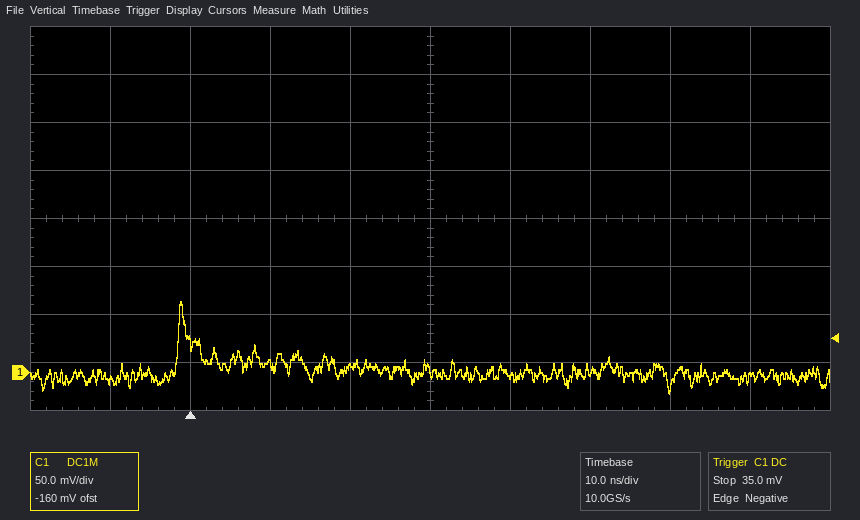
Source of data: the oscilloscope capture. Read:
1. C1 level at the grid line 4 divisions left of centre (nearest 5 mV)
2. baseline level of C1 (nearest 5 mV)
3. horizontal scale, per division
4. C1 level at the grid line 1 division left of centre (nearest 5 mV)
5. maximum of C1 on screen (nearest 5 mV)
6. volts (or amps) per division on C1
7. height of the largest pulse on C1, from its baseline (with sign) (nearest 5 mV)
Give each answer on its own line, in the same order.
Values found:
-10 mV
0 mV
10 ns
5 mV
75 mV
50 mV
+75 mV
